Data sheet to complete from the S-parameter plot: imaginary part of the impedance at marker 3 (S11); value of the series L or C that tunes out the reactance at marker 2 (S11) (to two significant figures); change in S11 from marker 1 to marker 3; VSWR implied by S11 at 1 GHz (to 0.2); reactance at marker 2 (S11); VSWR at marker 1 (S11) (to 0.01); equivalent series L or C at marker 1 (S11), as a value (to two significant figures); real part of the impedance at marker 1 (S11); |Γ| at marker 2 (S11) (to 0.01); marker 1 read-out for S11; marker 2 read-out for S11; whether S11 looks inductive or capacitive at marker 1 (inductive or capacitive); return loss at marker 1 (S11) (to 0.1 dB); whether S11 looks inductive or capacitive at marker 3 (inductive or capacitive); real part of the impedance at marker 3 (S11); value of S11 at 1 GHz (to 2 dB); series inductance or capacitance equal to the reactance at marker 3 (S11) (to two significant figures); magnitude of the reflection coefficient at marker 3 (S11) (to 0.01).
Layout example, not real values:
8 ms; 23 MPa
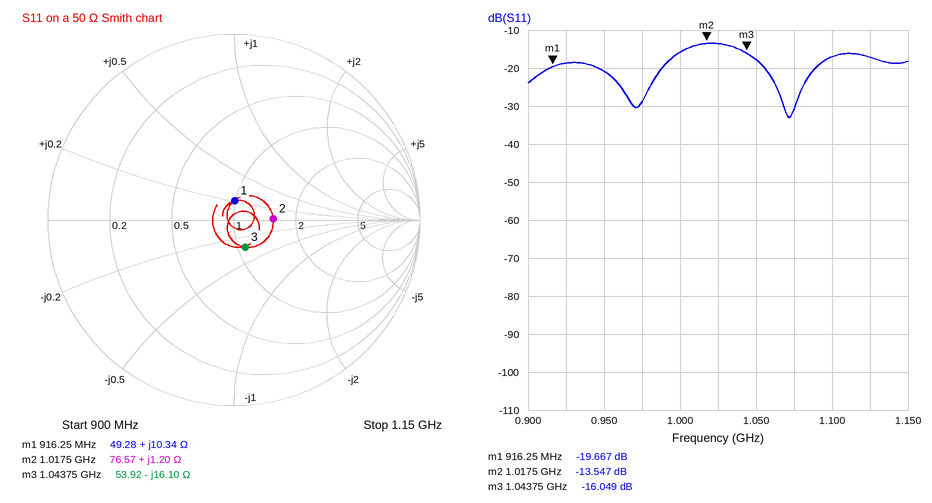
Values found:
-16.10 Ω; 130 pF; 3.618 dB; 1.4; +1.20 Ω; 1.23; 1.8 nH; 49.28 Ω; 0.21; -19.667 dB; -13.547 dB; inductive; 19.7 dB; capacitive; 53.92 Ω; -16 dB; 9.5 pF; 0.16
